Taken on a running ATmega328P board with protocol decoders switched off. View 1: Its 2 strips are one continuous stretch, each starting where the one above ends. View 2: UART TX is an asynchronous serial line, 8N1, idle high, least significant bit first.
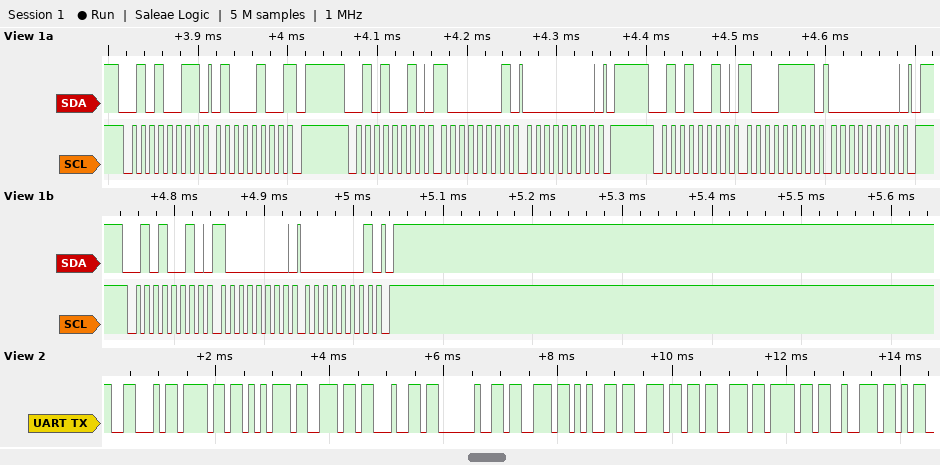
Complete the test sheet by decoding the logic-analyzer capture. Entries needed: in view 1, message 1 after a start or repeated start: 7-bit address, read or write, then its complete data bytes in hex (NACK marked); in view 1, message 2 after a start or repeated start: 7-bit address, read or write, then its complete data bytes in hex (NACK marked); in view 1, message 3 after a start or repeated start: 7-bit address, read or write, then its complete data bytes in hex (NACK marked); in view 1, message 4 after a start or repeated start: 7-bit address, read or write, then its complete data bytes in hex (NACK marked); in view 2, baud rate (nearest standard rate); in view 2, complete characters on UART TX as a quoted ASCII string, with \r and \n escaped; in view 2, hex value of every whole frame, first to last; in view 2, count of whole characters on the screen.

0x29 read: 44 NACK
0x29 write: 81 00
0x29 write: 8F 00
0x29 write: 80 01
9600 baud
"Found sensor"
46 6F 75 6E 64 20 73 65 6E 73 6F 72
12
